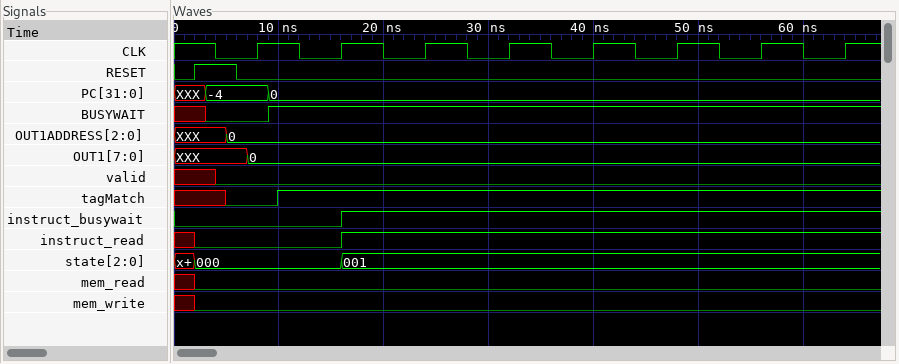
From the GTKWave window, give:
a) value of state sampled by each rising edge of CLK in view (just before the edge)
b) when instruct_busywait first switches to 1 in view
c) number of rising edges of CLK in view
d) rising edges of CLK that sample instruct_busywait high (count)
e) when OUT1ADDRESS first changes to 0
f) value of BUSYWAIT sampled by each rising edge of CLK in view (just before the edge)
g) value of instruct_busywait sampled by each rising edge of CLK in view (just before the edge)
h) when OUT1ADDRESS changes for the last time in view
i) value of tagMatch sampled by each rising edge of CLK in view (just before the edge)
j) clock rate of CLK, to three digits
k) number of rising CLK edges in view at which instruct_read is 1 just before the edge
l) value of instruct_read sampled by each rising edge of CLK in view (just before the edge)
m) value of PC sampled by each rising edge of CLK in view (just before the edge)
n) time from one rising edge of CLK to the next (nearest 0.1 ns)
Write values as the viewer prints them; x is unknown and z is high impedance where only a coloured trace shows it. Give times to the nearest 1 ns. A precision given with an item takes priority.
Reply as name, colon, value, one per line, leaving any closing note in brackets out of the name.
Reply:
value of state sampled by each rising edge of CLK in view: 000, 000, 001, 001, 001, 001, 001, 001
when instruct_busywait first switches to 1 in view: 16 ns
number of rising edges of CLK in view: 8
rising edges of CLK that sample instruct_busywait high: 6
when OUT1ADDRESS first changes to 0: 5 ns
value of BUSYWAIT sampled by each rising edge of CLK in view: 0 1 1 1 1 1 1 1
value of instruct_busywait sampled by each rising edge of CLK in view: 0 0 1 1 1 1 1 1
when OUT1ADDRESS changes for the last time in view: 5 ns
value of tagMatch sampled by each rising edge of CLK in view: 0 1 1 1 1 1 1 1
clock rate of CLK, to three digits: 125 MHz
number of rising CLK edges in view at which instruct_read is 1 just before the edge: 6
value of instruct_read sampled by each rising edge of CLK in view: 0 0 1 1 1 1 1 1
value of PC sampled by each rising edge of CLK in view: -4, 0, 0, 0, 0, 0, 0, 0
time from one rising edge of CLK to the next: 8 ns
